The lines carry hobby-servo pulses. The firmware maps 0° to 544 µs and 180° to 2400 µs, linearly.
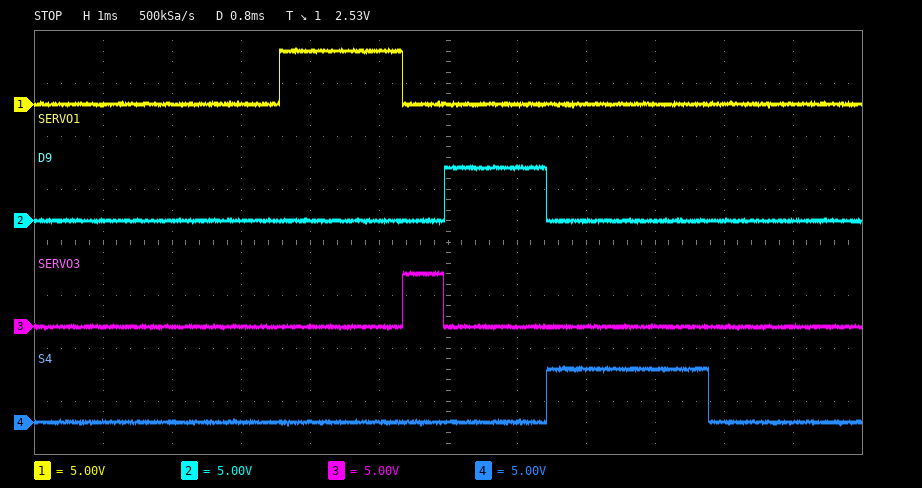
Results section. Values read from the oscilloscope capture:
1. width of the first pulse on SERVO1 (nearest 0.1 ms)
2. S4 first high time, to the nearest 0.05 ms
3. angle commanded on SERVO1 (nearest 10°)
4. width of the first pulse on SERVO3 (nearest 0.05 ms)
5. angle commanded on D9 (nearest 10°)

1.8 ms
2.35 ms
120°
0.60 ms
90°
